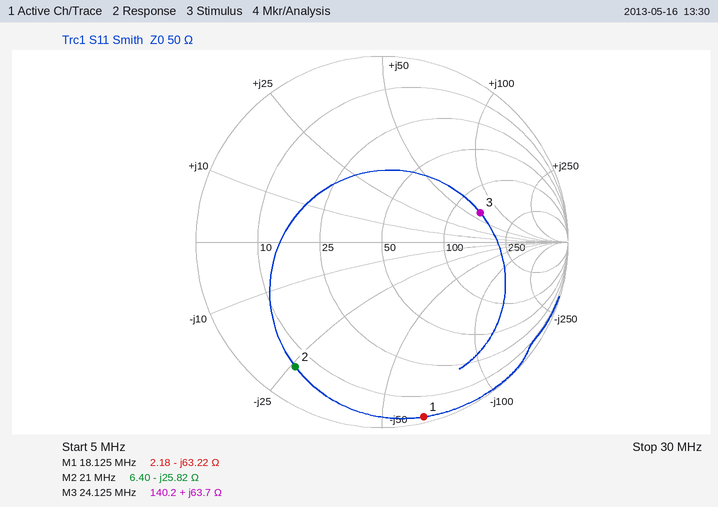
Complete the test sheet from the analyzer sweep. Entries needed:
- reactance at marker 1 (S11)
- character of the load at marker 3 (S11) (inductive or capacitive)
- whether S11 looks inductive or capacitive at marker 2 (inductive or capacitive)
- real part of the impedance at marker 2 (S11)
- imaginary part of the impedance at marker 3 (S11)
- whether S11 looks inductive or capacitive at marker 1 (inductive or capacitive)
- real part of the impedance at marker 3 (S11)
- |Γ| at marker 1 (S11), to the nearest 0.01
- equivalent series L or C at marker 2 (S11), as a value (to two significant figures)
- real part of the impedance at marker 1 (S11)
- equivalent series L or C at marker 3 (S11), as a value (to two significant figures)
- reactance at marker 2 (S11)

-63.22 Ω
inductive
capacitive
6.40 Ω
+63.7 Ω
capacitive
140.2 Ω
0.97
290 pF
2.18 Ω
420 nH
-25.82 Ω
